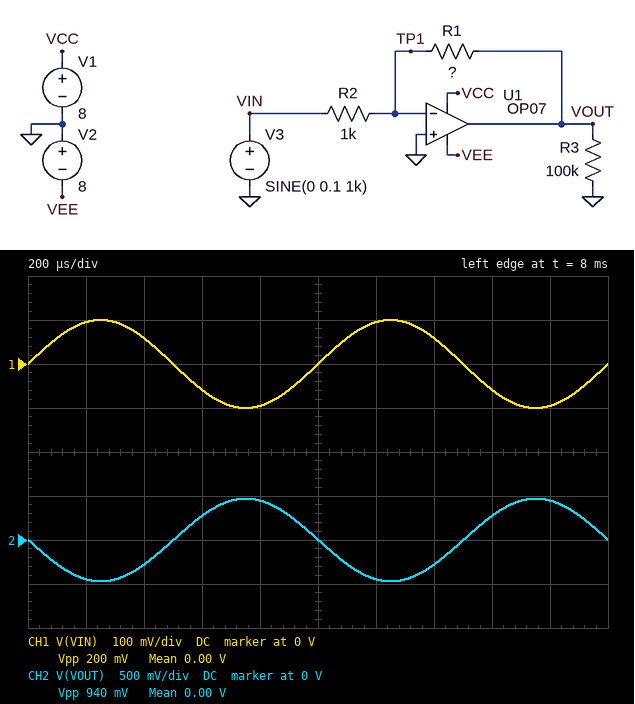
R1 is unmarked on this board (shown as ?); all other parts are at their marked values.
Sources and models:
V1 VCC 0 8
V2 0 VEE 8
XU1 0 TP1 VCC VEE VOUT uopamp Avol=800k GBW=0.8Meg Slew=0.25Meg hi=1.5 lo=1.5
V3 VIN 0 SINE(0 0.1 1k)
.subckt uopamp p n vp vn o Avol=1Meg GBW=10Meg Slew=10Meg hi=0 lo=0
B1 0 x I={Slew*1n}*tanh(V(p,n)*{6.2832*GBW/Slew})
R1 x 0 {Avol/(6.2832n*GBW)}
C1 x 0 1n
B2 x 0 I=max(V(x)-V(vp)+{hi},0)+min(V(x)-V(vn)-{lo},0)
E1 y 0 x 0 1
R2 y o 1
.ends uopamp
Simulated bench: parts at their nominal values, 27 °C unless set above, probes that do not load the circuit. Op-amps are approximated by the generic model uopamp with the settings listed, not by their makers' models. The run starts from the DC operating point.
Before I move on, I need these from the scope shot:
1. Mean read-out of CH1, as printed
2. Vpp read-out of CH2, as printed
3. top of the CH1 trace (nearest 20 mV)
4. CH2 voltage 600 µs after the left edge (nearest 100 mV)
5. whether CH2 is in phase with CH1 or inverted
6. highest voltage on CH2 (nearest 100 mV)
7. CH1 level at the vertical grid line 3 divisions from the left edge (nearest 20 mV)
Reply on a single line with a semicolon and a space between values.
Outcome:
0.00 V; 940 mV; 100 mV; 300 mV; inverted; 500 mV; -60 mV
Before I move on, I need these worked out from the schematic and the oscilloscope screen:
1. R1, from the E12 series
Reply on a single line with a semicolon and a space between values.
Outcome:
4.7 kΩ
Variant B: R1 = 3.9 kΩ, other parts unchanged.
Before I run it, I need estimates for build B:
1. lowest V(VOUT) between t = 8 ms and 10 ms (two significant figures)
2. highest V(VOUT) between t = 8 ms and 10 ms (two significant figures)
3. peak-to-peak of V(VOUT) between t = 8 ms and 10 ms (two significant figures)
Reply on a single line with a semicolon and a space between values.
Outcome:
-390 mV; 390 mV; 780 mV
